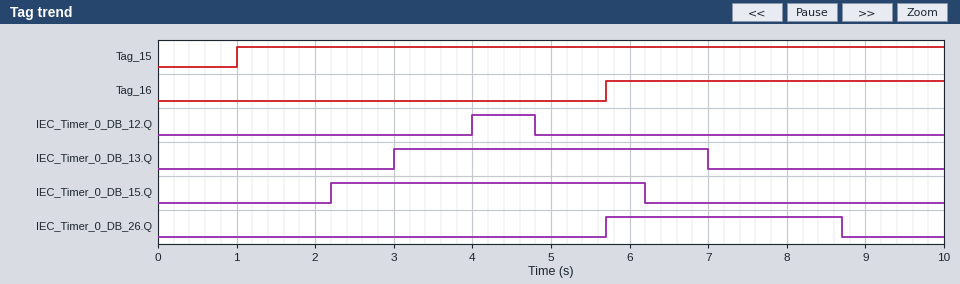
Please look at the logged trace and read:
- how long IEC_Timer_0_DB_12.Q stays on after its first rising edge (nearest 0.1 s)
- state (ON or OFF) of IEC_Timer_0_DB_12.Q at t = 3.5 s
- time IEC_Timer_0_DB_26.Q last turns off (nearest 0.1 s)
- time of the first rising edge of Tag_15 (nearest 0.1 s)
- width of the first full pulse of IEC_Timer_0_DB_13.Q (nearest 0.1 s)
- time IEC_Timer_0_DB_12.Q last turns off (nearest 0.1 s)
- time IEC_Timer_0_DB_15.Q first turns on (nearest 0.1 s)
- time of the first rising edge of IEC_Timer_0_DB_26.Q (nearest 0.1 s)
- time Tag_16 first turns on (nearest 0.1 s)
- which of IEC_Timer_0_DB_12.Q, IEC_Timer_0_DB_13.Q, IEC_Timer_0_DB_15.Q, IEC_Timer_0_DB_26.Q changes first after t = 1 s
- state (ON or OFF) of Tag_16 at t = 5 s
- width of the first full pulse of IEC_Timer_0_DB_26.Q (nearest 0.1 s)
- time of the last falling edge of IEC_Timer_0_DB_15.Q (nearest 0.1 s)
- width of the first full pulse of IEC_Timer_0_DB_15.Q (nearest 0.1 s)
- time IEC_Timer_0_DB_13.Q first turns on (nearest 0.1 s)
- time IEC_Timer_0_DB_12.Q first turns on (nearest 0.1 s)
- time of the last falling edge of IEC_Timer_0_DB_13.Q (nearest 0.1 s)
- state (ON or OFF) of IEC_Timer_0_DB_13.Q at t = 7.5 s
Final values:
0.8 s
OFF
8.7 s
1.0 s
4.0 s
4.8 s
2.2 s
5.7 s
5.7 s
IEC_Timer_0_DB_15.Q
OFF
3.0 s
6.2 s
4.0 s
3.0 s
4.0 s
7.0 s
OFF
